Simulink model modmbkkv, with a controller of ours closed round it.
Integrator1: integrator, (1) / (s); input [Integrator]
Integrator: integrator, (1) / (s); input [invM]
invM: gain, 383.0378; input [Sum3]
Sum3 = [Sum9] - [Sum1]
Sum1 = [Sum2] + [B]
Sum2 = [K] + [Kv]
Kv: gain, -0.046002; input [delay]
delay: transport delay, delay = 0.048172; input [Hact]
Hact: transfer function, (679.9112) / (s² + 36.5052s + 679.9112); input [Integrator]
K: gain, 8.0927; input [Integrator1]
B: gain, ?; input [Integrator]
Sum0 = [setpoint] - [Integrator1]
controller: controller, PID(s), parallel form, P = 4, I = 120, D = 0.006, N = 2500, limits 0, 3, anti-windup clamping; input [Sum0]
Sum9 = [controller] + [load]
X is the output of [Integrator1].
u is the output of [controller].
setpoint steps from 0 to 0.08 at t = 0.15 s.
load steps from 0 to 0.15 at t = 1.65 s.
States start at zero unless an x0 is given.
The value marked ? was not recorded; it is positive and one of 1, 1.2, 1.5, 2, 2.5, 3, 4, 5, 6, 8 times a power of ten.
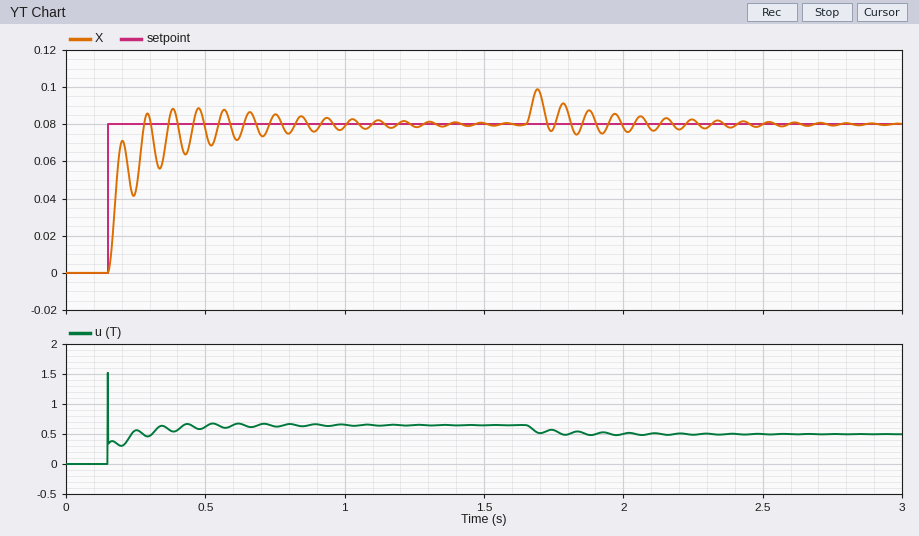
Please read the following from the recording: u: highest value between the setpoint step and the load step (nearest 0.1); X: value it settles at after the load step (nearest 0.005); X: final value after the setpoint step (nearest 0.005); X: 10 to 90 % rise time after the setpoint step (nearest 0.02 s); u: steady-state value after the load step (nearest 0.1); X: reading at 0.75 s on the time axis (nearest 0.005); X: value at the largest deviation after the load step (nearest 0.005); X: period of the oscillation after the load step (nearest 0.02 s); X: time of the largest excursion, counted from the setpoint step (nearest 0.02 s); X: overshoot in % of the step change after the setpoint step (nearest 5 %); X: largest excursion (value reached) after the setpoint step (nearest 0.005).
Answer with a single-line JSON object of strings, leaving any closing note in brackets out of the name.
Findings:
{"u: highest value between the setpoint step and the load step": "1.5", "X: value it settles at after the load step": "0.080", "X: final value after the setpoint step": "0.080", "X: 10 to 90 % rise time after the setpoint step": "0.12 s", "u: steady-state value after the load step": "0.5", "X: reading at 0.75 s on the time axis": "0.085", "X: value at the largest deviation after the load step": "0.100", "X: period of the oscillation after the load step": "0.10 s", "X: time of the largest excursion, counted from the setpoint step": "0.32 s", "X: overshoot in % of the step change after the setpoint step": "10 %", "X: largest excursion (value reached) after the setpoint step": "0.090"}
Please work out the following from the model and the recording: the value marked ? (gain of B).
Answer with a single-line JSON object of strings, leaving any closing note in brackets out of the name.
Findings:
{"the value marked ?": "0.04"}
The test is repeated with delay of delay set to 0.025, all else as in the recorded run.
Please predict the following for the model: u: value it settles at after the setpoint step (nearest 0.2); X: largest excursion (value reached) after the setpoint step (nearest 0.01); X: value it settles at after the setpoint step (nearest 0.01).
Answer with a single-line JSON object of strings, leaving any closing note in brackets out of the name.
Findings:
{"u: value it settles at after the setpoint step": "0.6", "X: largest excursion (value reached) after the setpoint step": "0.08", "X: value it settles at after the setpoint step": "0.08"}
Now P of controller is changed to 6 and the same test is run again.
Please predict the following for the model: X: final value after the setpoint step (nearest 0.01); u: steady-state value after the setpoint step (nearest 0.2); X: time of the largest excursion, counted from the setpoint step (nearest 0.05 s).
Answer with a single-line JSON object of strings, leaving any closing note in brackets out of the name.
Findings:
{"X: final value after the setpoint step": "0.08", "u: steady-state value after the setpoint step": "0.6", "X: time of the largest excursion, counted from the setpoint step": "0.20 s"}
